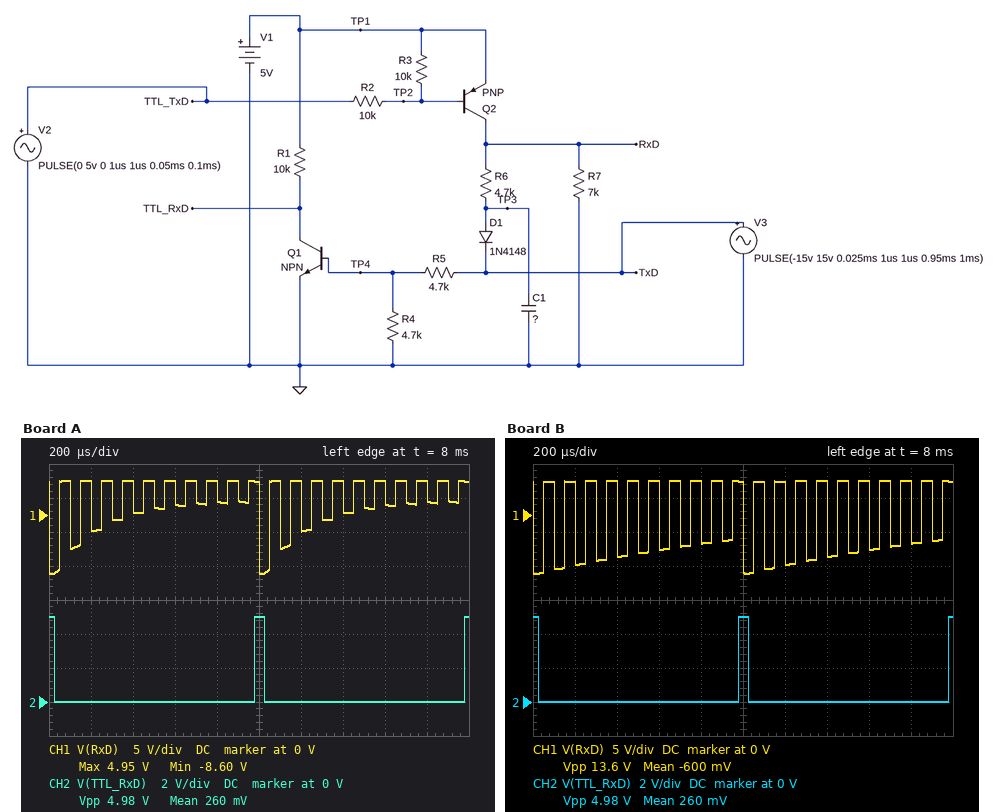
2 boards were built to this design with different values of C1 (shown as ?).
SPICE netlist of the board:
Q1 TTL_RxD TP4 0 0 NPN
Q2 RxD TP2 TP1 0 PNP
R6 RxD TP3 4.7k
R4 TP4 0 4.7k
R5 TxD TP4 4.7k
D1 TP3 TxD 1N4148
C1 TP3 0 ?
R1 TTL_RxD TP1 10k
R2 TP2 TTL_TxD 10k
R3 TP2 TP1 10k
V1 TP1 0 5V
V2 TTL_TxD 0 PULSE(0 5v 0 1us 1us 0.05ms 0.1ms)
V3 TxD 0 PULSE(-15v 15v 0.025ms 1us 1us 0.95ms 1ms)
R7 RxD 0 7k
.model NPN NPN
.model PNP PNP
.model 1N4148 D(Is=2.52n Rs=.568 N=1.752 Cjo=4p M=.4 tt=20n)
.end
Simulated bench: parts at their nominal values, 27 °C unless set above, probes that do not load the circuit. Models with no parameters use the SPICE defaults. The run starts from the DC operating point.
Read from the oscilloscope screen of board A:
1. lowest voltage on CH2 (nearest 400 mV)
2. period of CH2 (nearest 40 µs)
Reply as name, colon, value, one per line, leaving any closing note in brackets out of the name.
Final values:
lowest voltage on CH2: 0 V
period of CH2: 1.00 ms
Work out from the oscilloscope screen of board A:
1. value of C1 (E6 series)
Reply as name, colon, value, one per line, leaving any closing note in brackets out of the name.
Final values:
value of C1: 33 nF
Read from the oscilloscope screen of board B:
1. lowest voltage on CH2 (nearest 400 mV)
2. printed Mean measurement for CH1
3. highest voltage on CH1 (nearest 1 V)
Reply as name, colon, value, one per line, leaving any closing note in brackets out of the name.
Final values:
lowest voltage on CH2: 0 V
printed Mean measurement for CH1: -600 mV
highest voltage on CH1: 5 V
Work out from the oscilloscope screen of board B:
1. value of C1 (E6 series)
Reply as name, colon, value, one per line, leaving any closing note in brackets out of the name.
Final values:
value of C1: 220 nF
